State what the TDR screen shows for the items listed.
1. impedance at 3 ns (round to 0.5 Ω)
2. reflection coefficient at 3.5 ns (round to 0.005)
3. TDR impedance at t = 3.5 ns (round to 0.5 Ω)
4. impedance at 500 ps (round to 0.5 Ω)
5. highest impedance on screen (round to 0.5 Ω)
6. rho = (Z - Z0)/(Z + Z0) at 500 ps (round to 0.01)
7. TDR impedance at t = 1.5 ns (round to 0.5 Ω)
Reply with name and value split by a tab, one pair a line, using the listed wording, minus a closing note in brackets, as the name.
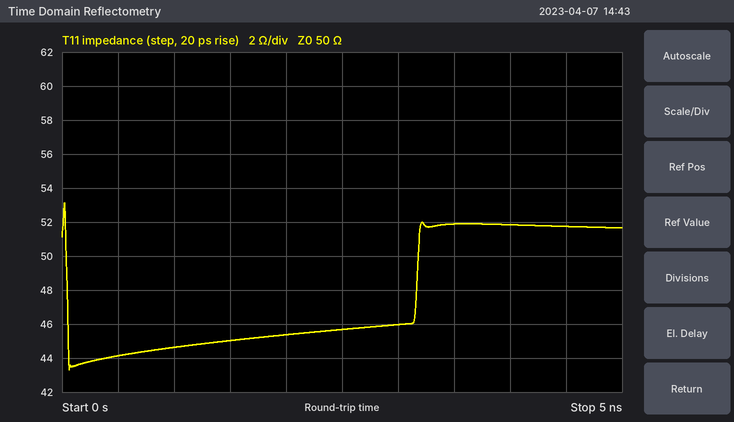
impedance at 3 ns	46.0 Ω
reflection coefficient at 3.5 ns	+0.020
TDR impedance at t = 3.5 ns	52.0 Ω
impedance at 500 ps	44.0 Ω
highest impedance on screen	53.0 Ω
rho = (Z - Z0)/(Z + Z0) at 500 ps	-0.06
TDR impedance at t = 1.5 ns	45.0 Ω
